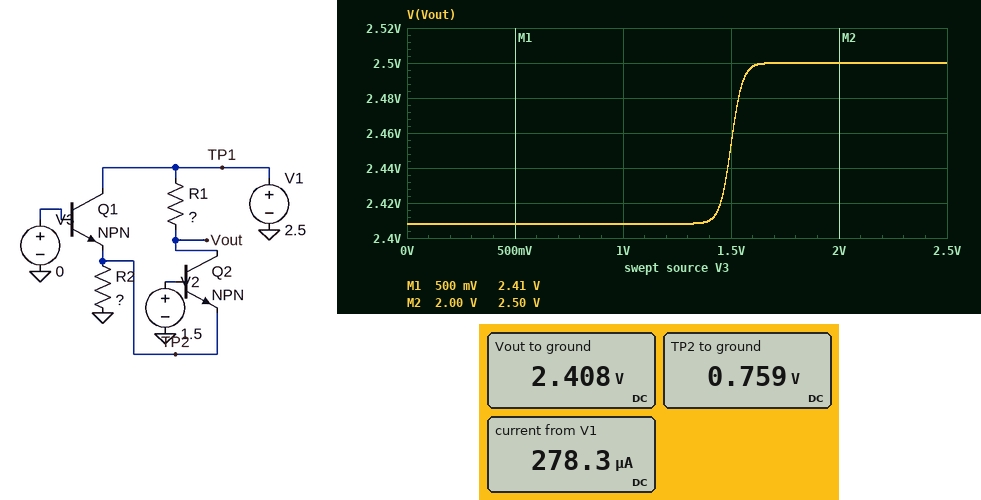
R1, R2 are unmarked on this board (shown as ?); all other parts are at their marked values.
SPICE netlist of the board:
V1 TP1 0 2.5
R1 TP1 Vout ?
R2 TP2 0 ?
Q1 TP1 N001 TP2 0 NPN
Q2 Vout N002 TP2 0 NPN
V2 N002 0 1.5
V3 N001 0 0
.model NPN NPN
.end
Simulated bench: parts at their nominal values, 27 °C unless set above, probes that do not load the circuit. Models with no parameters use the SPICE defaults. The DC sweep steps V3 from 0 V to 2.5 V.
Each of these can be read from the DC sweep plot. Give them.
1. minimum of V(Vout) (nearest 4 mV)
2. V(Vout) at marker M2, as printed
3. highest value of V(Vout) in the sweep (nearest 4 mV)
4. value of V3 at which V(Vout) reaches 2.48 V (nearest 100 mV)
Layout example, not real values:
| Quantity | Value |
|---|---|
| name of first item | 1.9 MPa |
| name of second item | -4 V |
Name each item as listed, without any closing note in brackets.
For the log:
| Quantity | Value |
|---|---|
| minimum of V(Vout) | 2.408 V |
| V(Vout) at marker M2, as printed | 2.50 V |
| highest value of V(Vout) in the sweep | 2.500 V |
| value of V3 at which V(Vout) reaches 2.48 V | 1.5 V |
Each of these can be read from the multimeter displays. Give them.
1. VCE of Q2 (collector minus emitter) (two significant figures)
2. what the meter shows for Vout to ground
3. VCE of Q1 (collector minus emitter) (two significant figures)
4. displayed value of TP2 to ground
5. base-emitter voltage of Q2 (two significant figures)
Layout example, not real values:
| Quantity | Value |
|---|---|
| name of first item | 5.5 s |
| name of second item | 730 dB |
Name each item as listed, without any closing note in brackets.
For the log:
| Quantity | Value |
|---|---|
| VCE of Q2 (collector minus emitter) | 1.6 V |
| what the meter shows for Vout to ground | 2.408 V |
| VCE of Q1 (collector minus emitter) | 1.7 V |
| displayed value of TP2 to ground | 0.759 V |
| base-emitter voltage of Q2 | 740 mV |
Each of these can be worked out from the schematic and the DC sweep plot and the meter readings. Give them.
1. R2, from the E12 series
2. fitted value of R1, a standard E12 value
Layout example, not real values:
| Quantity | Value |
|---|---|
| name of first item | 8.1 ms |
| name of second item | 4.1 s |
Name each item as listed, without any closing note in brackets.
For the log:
| Quantity | Value |
|---|---|
| R2, from the E12 series | 2.7 kΩ |
| fitted value of R1, a standard E12 value | 330 Ω |
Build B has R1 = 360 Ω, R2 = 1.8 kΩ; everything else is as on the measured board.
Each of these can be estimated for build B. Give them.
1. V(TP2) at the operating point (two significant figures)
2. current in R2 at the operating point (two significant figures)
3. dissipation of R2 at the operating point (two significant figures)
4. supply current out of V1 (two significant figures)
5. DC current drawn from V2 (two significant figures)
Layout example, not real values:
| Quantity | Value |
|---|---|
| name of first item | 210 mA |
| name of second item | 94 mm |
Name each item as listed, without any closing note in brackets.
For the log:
| Quantity | Value |
|---|---|
| V(TP2) at the operating point | 750 mV |
| current in R2 at the operating point | 420 µA |
| dissipation of R2 at the operating point | 310 µW |
| supply current out of V1 | 410 µA |
| DC current drawn from V2 | 4.1 µA |
